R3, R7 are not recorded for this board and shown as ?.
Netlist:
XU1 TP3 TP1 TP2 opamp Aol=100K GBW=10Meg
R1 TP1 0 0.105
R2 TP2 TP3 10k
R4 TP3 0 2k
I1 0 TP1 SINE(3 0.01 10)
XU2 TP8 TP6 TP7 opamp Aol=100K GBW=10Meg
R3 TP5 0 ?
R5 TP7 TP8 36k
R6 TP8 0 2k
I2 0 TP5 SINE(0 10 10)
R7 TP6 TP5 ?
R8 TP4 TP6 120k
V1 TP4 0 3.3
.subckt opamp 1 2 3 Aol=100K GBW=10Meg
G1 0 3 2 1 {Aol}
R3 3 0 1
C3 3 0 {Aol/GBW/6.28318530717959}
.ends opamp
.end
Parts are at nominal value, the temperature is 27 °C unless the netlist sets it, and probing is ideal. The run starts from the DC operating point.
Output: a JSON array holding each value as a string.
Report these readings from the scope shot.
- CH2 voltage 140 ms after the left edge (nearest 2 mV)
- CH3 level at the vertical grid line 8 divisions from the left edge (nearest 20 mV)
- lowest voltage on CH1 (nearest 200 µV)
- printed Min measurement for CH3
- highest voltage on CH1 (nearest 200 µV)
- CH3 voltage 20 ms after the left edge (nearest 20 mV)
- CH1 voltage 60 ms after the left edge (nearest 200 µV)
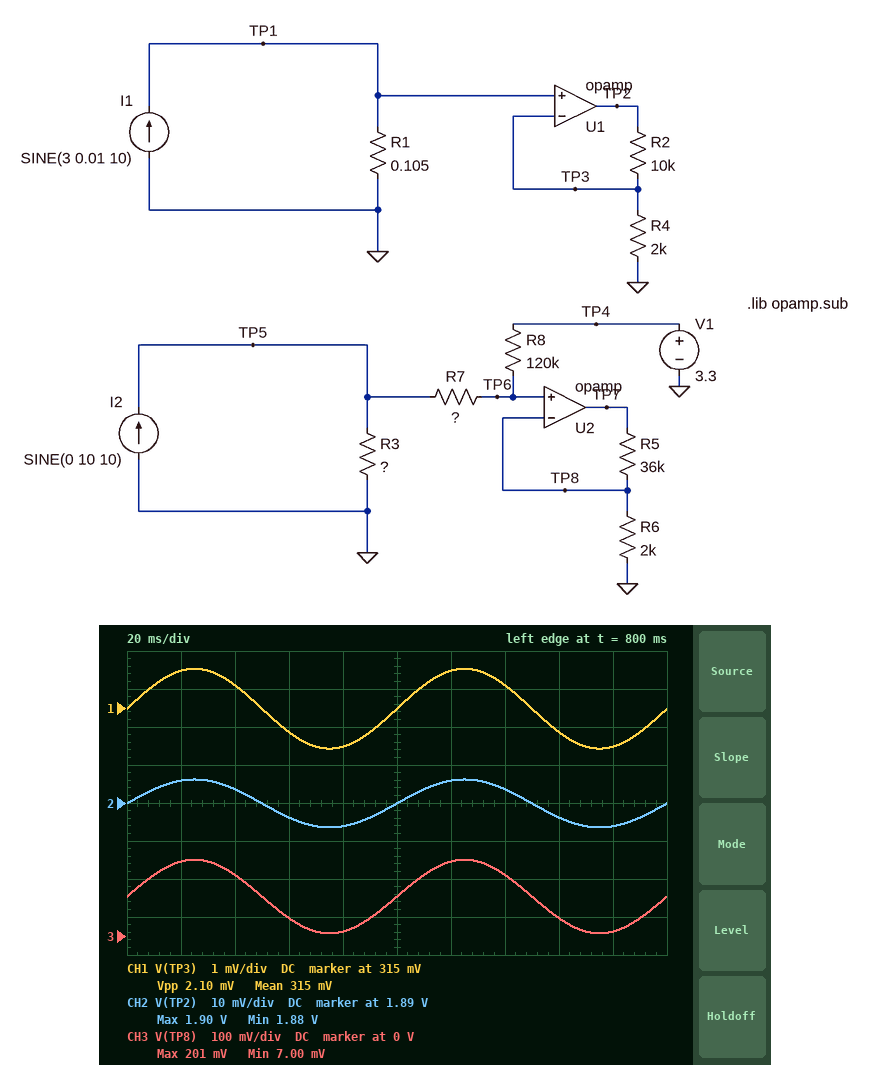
["1.894 V", "40 mV", "314.0 mV", "7.00 mV", "316.0 mV", "200 mV", "314.4 mV"]
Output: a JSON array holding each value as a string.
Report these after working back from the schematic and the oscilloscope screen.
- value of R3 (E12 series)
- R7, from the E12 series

["0.01 Ω", "3.9 kΩ"]
